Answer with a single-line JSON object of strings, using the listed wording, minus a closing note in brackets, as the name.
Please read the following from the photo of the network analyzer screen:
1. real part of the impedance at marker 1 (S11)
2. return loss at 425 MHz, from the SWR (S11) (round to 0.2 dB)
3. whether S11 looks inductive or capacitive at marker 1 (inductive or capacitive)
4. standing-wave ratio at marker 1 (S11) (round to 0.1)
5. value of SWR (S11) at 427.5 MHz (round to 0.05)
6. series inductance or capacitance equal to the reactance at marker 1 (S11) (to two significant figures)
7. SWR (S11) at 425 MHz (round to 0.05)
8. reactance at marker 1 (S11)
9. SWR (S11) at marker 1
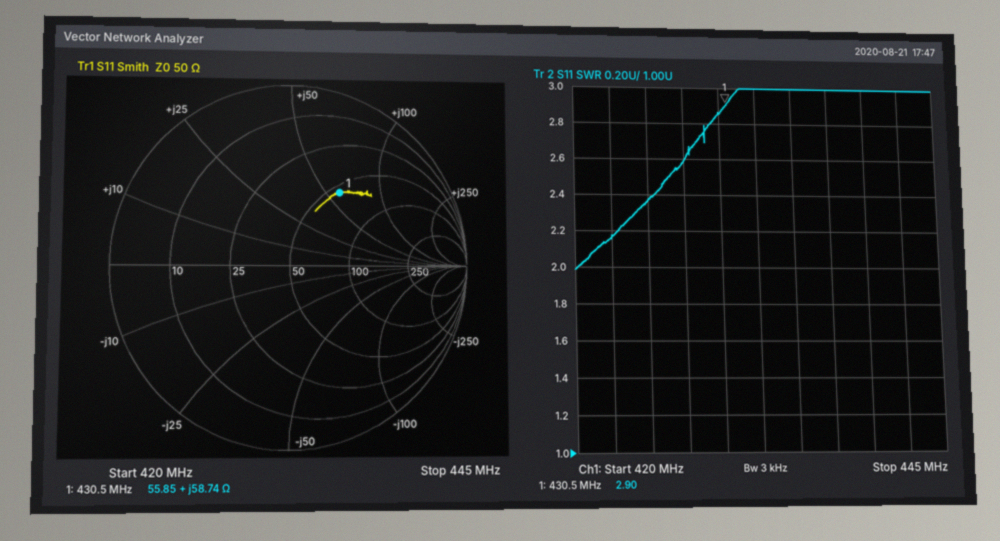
{"real part of the impedance at marker 1": "55.85 Ω", "return loss at 425 MHz, from the SWR (S11)": "7.8 dB", "whether S11 looks inductive or capacitive at marker 1": "inductive", "standing-wave ratio at marker 1 (S11)": "2.9", "value of SWR (S11) at 427.5 MHz": "2.60", "series inductance or capacitance equal to the reactance at marker 1 (S11)": "22 nH", "SWR (S11) at 425 MHz": "2.35", "reactance at marker 1": "+58.74 Ω", "SWR (S11) at marker 1": "2.90"}
